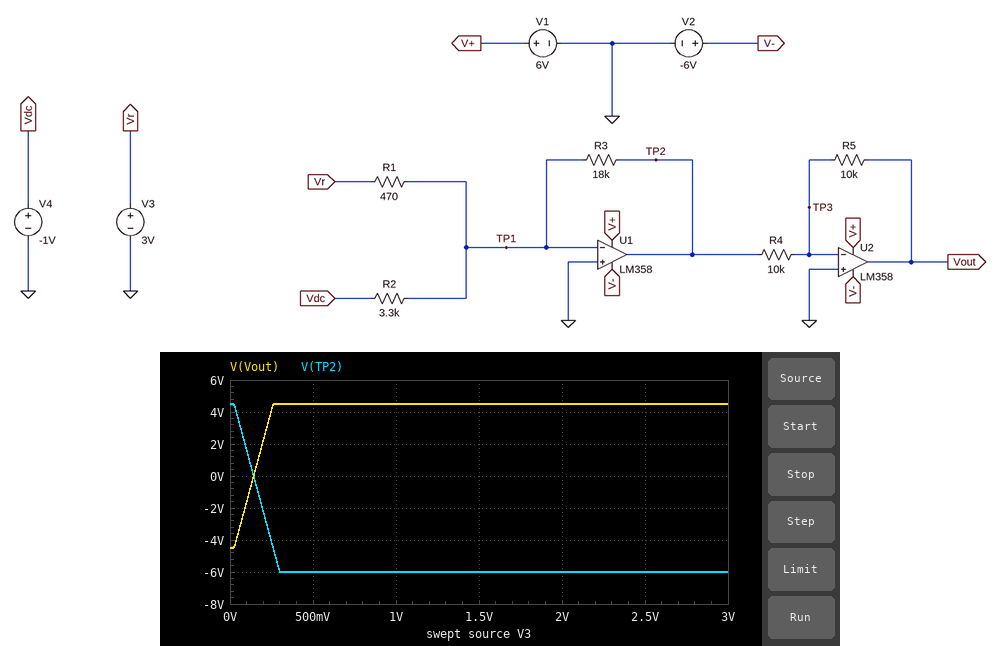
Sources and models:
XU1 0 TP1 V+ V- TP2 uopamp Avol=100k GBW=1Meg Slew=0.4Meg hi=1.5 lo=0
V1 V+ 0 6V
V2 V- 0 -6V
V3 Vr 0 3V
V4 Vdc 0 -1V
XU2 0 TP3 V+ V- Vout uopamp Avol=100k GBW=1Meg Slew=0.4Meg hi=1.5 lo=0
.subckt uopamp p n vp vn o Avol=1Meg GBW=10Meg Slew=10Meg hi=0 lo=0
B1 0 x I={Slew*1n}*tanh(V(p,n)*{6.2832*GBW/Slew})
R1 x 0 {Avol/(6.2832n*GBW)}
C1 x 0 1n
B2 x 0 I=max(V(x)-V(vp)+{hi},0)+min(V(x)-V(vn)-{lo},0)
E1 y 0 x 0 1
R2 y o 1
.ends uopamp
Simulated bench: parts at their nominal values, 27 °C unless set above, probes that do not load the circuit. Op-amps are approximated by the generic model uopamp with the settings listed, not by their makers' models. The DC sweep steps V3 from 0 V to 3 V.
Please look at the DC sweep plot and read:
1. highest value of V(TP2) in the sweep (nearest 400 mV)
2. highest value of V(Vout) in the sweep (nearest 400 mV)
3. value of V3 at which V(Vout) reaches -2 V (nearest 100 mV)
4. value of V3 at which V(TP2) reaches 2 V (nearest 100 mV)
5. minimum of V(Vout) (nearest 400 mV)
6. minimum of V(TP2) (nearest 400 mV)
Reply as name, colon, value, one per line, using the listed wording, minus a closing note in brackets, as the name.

highest value of V(TP2) in the sweep: 4.4 V
highest value of V(Vout) in the sweep: 4.4 V
value of V3 at which V(Vout) reaches -2 V: 100 mV
value of V3 at which V(TP2) reaches 2 V: 100 mV
minimum of V(Vout): -4.4 V
minimum of V(TP2): -6.0 V
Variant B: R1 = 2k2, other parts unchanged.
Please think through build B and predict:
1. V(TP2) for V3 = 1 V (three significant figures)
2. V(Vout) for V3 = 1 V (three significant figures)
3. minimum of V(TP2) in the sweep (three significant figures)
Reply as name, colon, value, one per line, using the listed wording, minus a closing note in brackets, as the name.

V(TP2) for V3 = 1 V: -2.73 V
V(Vout) for V3 = 1 V: 2.73 V
minimum of V(TP2) in the sweep: -6.00 V
